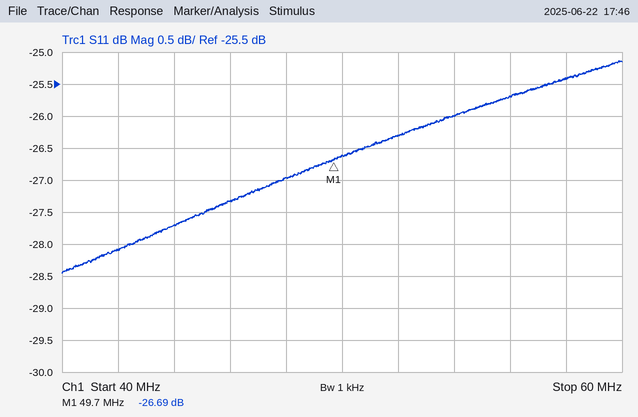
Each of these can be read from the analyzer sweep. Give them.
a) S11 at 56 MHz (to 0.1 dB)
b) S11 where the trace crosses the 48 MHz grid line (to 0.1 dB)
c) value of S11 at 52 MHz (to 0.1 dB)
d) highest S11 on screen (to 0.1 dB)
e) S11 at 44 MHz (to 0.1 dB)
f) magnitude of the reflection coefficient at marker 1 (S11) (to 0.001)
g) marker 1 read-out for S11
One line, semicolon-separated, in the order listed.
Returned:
-25.7 dB; -27.0 dB; -26.3 dB; -25.1 dB; -27.7 dB; 0.046; -26.69 dB
